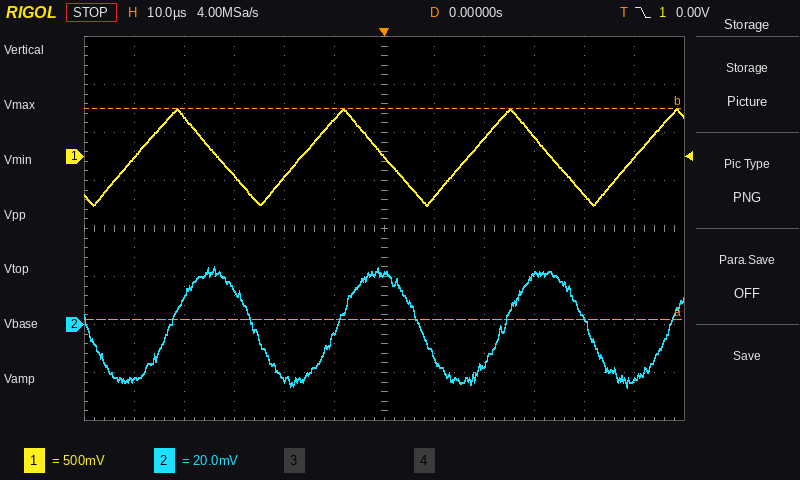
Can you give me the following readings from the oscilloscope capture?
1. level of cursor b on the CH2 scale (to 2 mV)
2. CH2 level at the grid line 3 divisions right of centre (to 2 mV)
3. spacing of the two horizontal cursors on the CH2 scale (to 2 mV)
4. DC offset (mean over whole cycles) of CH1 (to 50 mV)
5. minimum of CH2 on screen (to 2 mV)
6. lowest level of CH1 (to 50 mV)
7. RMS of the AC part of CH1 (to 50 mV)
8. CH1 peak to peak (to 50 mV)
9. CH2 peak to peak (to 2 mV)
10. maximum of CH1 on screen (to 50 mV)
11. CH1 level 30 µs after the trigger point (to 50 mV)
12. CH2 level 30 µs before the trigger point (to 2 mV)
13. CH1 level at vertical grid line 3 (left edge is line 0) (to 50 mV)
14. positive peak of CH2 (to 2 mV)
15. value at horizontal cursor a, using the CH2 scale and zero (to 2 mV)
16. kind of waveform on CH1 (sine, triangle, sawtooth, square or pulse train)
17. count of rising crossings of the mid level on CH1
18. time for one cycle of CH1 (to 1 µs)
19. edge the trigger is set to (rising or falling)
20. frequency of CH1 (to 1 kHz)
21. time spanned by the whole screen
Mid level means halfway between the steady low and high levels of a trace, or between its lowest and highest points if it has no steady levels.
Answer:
90 mV
20 mV
88 mV
0 mV
-26 mV
-500 mV
300 mV
1.00 V
50 mV
500 mV
200 mV
14 mV
-200 mV
24 mV
2 mV
triangle
4
33 µs
falling
30 kHz
120 µs
